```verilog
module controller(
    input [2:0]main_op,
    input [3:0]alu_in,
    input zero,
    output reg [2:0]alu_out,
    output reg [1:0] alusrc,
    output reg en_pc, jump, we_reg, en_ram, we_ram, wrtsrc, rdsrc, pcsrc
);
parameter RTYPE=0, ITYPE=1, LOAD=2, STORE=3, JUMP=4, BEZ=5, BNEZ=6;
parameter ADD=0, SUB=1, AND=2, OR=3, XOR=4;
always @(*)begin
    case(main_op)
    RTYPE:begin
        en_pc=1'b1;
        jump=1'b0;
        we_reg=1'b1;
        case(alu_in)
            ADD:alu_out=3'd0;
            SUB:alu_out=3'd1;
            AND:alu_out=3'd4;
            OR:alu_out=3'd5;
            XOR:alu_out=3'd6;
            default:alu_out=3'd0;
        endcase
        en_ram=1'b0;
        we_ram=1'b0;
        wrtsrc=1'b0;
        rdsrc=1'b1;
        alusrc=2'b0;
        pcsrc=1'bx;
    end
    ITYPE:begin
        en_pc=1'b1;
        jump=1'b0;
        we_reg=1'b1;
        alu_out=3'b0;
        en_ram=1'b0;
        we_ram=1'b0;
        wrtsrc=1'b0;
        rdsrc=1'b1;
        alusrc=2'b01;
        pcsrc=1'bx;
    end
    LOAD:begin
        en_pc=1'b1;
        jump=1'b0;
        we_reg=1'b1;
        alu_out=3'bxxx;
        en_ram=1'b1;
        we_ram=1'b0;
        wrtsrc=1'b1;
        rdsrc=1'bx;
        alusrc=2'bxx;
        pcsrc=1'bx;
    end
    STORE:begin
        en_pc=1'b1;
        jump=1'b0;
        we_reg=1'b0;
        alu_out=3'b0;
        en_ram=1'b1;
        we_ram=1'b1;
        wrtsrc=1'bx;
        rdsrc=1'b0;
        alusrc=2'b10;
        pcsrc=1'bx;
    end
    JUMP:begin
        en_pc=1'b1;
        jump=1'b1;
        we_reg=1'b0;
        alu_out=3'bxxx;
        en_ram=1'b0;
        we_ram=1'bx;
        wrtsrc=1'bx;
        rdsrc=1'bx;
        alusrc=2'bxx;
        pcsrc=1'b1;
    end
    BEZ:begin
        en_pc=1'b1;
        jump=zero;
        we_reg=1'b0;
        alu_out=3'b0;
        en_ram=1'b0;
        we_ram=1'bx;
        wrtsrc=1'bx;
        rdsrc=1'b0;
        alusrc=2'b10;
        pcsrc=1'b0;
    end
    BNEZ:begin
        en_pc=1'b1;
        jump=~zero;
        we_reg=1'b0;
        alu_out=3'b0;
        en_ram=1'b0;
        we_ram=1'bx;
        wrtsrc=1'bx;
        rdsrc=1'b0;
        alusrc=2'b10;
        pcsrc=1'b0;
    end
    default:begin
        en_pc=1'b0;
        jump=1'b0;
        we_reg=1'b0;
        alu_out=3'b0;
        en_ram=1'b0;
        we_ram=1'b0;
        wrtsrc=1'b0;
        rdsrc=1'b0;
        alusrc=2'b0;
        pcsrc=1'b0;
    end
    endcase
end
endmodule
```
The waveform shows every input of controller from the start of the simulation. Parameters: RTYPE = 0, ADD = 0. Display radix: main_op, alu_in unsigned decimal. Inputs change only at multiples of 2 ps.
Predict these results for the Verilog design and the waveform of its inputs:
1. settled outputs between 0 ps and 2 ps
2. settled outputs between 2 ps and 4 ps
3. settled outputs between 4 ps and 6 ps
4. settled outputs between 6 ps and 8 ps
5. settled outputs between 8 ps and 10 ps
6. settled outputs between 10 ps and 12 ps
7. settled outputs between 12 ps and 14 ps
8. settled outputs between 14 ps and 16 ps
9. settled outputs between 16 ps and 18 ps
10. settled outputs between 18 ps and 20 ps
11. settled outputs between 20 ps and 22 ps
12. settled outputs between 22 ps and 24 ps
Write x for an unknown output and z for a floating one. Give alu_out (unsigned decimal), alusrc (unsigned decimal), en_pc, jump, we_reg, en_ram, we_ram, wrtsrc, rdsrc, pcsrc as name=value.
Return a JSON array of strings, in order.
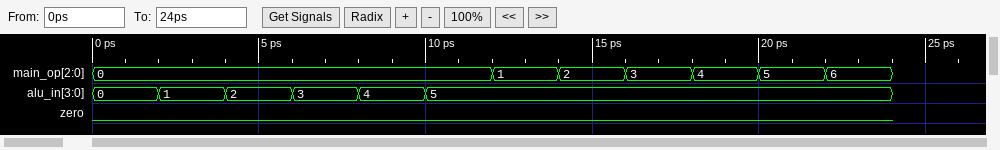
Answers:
["alu_out=0, alusrc=0, en_pc=1, jump=0, we_reg=1, en_ram=0, we_ram=0, wrtsrc=0, rdsrc=1, pcsrc=x", "alu_out=1, alusrc=0, en_pc=1, jump=0, we_reg=1, en_ram=0, we_ram=0, wrtsrc=0, rdsrc=1, pcsrc=x", "alu_out=4, alusrc=0, en_pc=1, jump=0, we_reg=1, en_ram=0, we_ram=0, wrtsrc=0, rdsrc=1, pcsrc=x", "alu_out=5, alusrc=0, en_pc=1, jump=0, we_reg=1, en_ram=0, we_ram=0, wrtsrc=0, rdsrc=1, pcsrc=x", "alu_out=6, alusrc=0, en_pc=1, jump=0, we_reg=1, en_ram=0, we_ram=0, wrtsrc=0, rdsrc=1, pcsrc=x", "alu_out=0, alusrc=0, en_pc=1, jump=0, we_reg=1, en_ram=0, we_ram=0, wrtsrc=0, rdsrc=1, pcsrc=x", "alu_out=0, alusrc=1, en_pc=1, jump=0, we_reg=1, en_ram=0, we_ram=0, wrtsrc=0, rdsrc=1, pcsrc=x", "alu_out=x, alusrc=x, en_pc=1, jump=0, we_reg=1, en_ram=1, we_ram=0, wrtsrc=1, rdsrc=x, pcsrc=x", "alu_out=0, alusrc=2, en_pc=1, jump=0, we_reg=0, en_ram=1, we_ram=1, wrtsrc=x, rdsrc=0, pcsrc=x", "alu_out=x, alusrc=x, en_pc=1, jump=1, we_reg=0, en_ram=0, we_ram=x, wrtsrc=x, rdsrc=x, pcsrc=1", "alu_out=0, alusrc=2, en_pc=1, jump=0, we_reg=0, en_ram=0, we_ram=x, wrtsrc=x, rdsrc=0, pcsrc=0", "alu_out=0, alusrc=2, en_pc=1, jump=1, we_reg=0, en_ram=0, we_ram=x, wrtsrc=x, rdsrc=0, pcsrc=0"]
